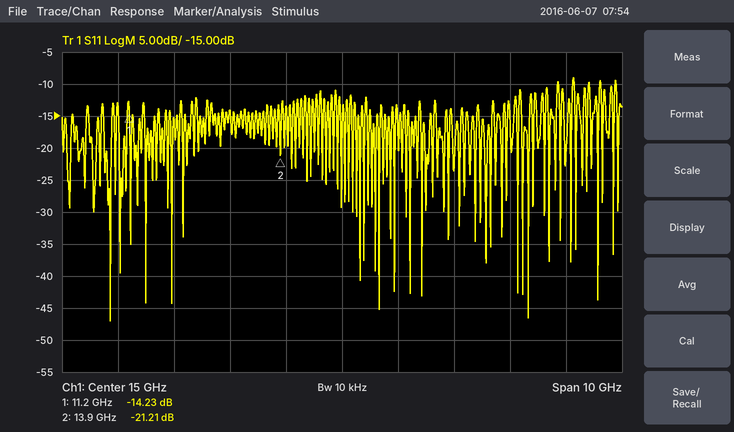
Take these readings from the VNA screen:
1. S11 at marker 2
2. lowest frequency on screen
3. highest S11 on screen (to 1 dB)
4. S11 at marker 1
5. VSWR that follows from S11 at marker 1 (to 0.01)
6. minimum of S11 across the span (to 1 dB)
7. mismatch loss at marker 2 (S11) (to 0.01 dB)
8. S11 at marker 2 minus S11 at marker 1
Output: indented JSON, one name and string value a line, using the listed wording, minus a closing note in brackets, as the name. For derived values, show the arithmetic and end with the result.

{
  "S11 at marker 2": "-21.21 dB",
  "lowest frequency on screen": "10 GHz",
  "highest S11 on screen": "-9 dB",
  "S11 at marker 1": "-14.23 dB",
  "VSWR that follows from S11 at marker 1": "(1 + 0.1943)/(1 − 0.1943) ≈ 1.48",
  "minimum of S11 across the span": "-47 dB",
  "mismatch loss at marker 2 (S11)": "−10 log10(1 − 10^(-21.21/10)) ≈ 0.03 dB",
  "S11 at marker 2 minus S11 at marker 1": "-21.21 − (-14.23) = -6.98 dB"
}
